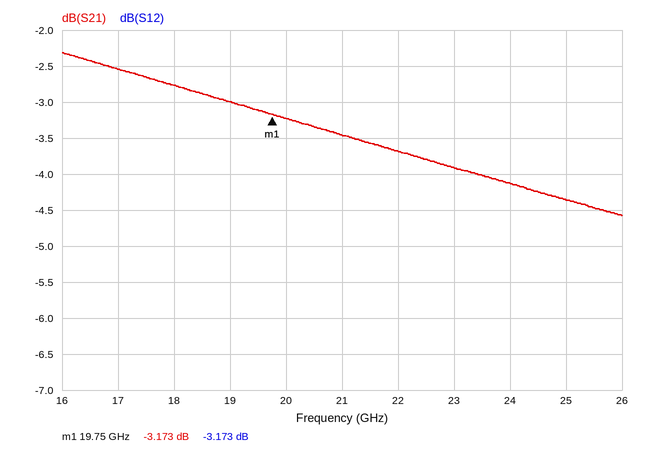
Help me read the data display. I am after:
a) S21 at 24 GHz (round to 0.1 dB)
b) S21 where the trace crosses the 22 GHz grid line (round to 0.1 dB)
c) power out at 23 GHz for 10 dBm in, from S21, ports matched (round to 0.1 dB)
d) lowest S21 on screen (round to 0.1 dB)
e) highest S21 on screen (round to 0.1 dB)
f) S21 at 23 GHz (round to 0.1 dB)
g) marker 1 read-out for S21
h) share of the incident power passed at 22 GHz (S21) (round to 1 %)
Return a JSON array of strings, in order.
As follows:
["-4.1 dB", "-3.7 dB", "6.1 dBm", "-4.6 dB", "-2.3 dB", "-3.9 dB", "-3.173 dB", "43 %"]
